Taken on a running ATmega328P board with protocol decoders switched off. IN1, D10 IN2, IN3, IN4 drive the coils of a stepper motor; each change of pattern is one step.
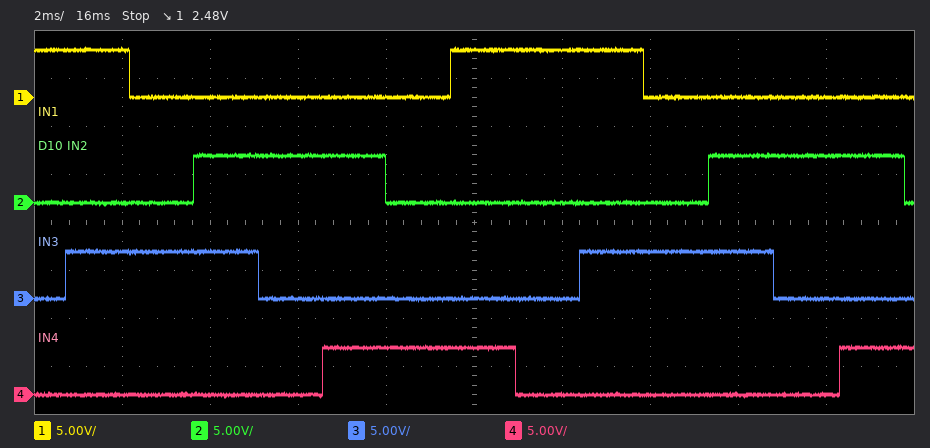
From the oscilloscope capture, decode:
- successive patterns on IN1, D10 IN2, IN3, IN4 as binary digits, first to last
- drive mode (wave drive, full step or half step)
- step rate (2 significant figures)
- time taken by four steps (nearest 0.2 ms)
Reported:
1000 1010 0010 0110 0100 0101 0001 1001 1000 1010 0010 0110 0100 0101 0001
half step
680 steps/s
5.8 ms
